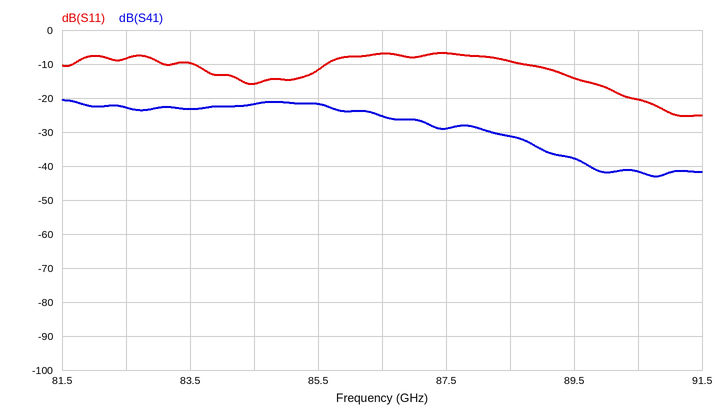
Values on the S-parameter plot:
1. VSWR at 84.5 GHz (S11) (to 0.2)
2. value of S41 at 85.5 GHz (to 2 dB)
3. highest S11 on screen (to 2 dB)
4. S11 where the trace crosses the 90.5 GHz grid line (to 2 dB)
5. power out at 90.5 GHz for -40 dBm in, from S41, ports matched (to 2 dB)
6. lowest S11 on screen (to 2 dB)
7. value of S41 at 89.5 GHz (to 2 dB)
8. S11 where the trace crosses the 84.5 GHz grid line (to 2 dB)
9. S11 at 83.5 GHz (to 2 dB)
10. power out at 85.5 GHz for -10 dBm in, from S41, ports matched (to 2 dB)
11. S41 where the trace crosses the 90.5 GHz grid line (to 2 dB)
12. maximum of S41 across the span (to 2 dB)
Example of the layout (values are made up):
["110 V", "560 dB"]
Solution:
["1.4", "-22 dB", "-6 dB", "-20 dB", "-82 dBm", "-26 dB", "-38 dB", "-16 dB", "-10 dB", "-32 dBm", "-42 dB", "-20 dB"]
